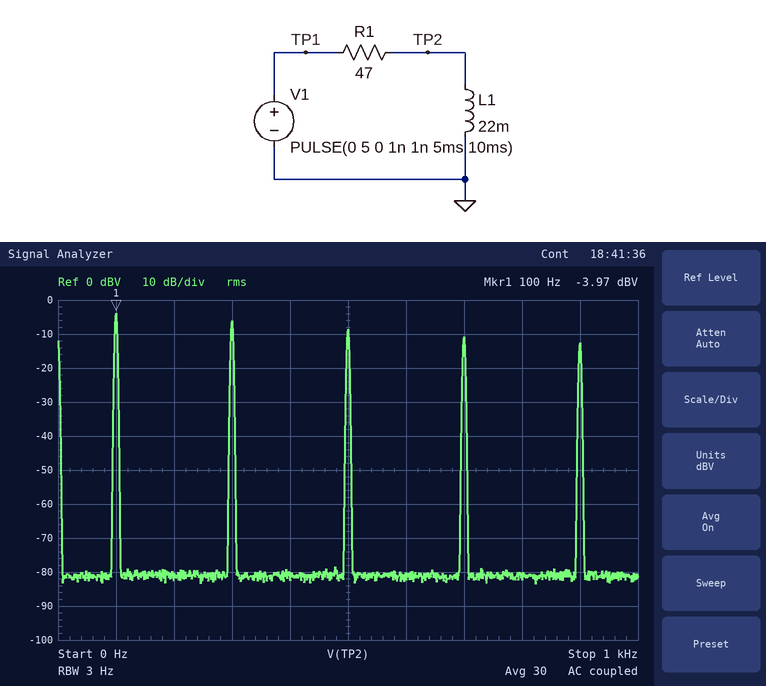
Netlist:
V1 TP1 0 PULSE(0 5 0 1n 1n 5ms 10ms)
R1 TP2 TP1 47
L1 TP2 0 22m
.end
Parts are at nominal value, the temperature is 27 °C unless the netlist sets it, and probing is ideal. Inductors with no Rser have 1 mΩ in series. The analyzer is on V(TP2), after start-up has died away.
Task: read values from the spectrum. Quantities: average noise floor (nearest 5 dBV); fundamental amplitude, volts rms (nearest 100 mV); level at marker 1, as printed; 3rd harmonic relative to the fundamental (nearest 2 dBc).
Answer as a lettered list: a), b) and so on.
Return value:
a) -80 dBV
b) 600 mV
c) -3.97 dBV
d) -2 dBc
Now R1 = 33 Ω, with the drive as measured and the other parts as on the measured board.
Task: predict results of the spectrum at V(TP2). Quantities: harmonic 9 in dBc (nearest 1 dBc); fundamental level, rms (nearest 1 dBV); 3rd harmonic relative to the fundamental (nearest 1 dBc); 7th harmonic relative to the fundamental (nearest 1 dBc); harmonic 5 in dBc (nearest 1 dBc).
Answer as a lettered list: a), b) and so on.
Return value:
a) -11 dBc
b) -1 dBV
c) -3 dBc
d) -9 dBc
e) -7 dBc
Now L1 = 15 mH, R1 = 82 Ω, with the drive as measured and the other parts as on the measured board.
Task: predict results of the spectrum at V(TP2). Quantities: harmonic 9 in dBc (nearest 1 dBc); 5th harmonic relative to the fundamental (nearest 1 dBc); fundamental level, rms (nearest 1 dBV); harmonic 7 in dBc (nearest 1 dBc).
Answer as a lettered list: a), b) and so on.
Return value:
a) -3 dBc
b) -1 dBc
c) -12 dBV
d) -2 dBc
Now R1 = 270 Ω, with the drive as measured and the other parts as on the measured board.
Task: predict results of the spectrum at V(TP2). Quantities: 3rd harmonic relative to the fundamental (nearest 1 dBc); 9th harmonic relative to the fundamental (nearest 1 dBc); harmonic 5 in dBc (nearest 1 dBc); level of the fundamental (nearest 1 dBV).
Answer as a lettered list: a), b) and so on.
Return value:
a) 0 dBc
b) -1 dBc
c) 0 dBc
d) -19 dBV
